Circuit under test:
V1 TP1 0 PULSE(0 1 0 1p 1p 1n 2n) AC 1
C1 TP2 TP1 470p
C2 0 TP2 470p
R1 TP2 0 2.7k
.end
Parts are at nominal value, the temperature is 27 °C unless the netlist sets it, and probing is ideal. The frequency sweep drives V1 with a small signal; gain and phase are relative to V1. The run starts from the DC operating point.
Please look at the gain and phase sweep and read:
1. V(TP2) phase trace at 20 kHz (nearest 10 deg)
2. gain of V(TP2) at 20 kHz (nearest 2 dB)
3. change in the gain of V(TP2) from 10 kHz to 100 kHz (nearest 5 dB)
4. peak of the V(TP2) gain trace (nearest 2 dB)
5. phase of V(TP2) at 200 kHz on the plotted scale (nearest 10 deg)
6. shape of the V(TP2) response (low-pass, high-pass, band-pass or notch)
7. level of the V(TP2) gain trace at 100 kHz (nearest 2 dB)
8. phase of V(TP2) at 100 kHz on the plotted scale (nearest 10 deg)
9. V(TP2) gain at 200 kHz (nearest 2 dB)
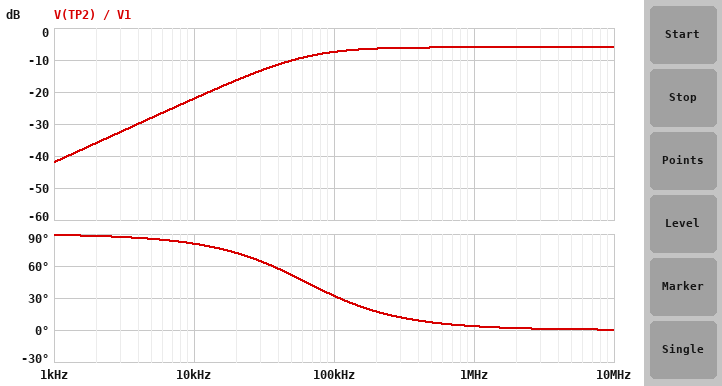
70 deg
-16 dB
15 dB
-6 dB
20 deg
high-pass
-8 dB
30 deg
-6 dB
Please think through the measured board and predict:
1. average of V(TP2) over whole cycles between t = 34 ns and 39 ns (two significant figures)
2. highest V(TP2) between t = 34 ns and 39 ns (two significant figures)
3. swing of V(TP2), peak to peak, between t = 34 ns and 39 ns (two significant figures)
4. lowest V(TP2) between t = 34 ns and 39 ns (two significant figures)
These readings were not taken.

250 mV
500 mV
500 mV
-3.7 mV
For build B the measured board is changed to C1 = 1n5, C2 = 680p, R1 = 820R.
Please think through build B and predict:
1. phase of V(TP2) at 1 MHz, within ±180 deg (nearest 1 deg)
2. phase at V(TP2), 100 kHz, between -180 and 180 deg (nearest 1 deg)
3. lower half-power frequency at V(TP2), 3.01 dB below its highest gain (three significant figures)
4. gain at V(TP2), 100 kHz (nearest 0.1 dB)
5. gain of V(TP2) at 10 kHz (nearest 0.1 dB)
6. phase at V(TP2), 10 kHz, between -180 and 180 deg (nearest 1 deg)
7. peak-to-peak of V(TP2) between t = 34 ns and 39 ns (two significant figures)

5 deg
42 deg
89.0 kHz
-5.8 dB
-22.3 dB
84 deg
690 mV
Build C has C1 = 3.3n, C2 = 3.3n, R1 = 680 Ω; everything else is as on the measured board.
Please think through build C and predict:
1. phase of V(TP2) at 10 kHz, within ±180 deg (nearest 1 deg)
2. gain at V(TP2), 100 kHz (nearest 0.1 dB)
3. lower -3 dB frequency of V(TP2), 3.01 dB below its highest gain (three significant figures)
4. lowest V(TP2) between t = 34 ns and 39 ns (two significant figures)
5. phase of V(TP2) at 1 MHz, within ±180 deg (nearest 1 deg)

74 deg
-6.5 dB
35.5 kHz
-2.1 mV
2 deg
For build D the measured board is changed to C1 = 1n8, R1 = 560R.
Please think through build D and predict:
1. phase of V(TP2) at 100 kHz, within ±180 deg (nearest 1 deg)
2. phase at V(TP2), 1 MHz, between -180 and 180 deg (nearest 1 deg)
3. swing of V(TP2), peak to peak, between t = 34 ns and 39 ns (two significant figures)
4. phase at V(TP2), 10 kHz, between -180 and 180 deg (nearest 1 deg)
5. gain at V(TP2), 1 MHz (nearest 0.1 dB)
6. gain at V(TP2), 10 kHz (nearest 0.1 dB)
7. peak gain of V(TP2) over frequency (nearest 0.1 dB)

51 deg
7 deg
790 mV
85 deg
-2.1 dB
-24.0 dB
-2.0 dB
